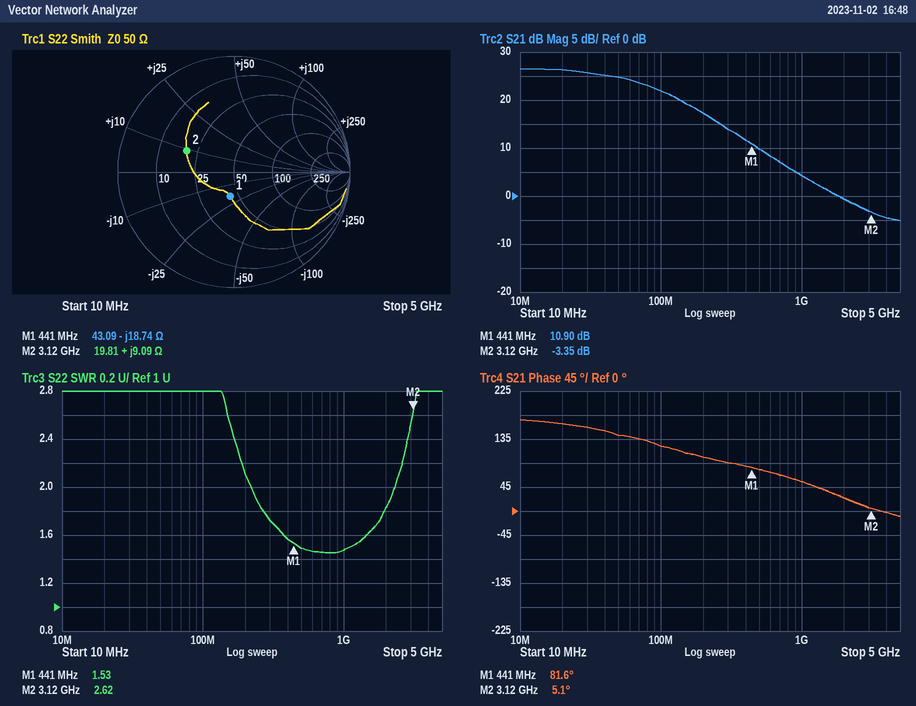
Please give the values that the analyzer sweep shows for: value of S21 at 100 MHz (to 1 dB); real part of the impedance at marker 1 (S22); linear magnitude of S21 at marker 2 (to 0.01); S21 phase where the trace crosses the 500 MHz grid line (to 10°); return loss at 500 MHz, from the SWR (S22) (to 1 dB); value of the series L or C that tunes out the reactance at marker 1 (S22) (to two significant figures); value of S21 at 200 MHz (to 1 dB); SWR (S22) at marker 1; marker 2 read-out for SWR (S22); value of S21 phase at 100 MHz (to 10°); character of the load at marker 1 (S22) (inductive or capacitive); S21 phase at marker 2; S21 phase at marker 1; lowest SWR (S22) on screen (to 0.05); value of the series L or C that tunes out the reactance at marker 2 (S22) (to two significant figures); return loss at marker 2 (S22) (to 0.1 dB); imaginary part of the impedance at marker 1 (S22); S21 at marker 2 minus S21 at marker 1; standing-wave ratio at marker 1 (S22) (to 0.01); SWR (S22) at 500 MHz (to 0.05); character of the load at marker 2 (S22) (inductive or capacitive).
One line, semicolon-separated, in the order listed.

22 dB; 43.09 Ω; 0.68; 80°; 14 dB; 6.8 nH; 17 dB; 1.53; 2.62; 120°; capacitive; 5.1°; 81.6°; 1.45; 5.6 pF; 7.0 dB; -18.74 Ω; -14.25 dB; 1.53; 1.50; inductive
